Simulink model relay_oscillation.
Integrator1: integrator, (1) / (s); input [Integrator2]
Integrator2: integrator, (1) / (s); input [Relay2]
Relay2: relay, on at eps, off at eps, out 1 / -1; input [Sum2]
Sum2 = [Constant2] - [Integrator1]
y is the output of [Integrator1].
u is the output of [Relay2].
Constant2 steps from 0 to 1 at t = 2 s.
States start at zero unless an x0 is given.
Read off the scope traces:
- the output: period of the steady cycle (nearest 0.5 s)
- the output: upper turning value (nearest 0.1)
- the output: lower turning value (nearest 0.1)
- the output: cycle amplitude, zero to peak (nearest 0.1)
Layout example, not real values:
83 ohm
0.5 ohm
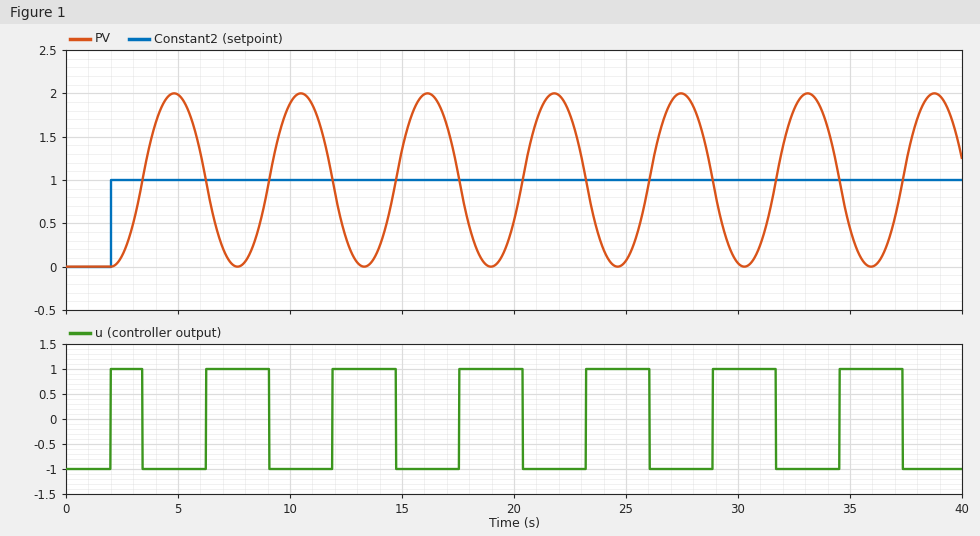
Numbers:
5.5 s
2.0
0.0
1.0
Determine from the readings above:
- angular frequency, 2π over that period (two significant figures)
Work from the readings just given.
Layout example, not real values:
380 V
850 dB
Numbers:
1.1 rad/s
